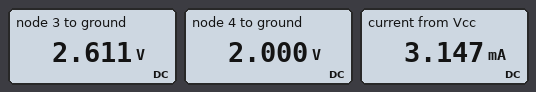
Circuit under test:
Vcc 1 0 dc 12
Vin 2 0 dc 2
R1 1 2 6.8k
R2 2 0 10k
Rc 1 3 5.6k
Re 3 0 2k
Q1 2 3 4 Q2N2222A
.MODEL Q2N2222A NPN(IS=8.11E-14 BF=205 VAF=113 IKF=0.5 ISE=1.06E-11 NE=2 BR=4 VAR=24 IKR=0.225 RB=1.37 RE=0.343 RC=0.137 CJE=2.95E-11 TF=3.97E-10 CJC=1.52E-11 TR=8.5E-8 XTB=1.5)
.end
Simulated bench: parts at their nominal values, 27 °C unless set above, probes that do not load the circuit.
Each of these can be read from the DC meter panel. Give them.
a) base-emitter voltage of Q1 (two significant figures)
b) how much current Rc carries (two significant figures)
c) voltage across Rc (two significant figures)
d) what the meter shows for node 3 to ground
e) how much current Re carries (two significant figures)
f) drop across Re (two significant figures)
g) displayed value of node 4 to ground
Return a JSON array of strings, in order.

["610 mV", "1.7 mA", "9.4 V", "2.611 V", "1.3 mA", "2.6 V", "2.000 V"]
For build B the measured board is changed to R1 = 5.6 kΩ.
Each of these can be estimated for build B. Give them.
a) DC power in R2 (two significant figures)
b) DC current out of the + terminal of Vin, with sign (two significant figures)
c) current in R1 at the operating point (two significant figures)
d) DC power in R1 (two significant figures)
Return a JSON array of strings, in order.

["400 µW", "-2.0 mA", "1.8 mA", "18 mW"]
